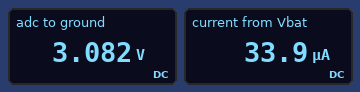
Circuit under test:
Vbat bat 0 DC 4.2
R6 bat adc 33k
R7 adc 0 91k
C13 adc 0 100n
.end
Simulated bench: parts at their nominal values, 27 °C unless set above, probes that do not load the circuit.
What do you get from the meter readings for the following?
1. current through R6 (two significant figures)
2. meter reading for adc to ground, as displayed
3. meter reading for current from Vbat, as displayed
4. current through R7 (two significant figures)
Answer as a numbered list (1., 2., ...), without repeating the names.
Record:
1. 34 µA
2. 3.082 V
3. 33.9 µA
4. 34 µA
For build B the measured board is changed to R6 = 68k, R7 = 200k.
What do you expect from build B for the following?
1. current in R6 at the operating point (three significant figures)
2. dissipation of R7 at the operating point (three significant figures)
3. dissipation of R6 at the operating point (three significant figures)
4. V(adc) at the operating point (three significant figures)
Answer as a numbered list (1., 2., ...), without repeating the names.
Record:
1. 15.7 µA
2. 49.1 µW
3. 16.7 µW
4. 3.13 V
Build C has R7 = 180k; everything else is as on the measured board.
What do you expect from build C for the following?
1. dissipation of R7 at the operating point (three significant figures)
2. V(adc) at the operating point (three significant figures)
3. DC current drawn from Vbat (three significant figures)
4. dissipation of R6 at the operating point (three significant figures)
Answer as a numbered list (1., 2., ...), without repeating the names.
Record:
1. 70.0 µW
2. 3.55 V
3. 19.7 µA
4. 12.8 µW
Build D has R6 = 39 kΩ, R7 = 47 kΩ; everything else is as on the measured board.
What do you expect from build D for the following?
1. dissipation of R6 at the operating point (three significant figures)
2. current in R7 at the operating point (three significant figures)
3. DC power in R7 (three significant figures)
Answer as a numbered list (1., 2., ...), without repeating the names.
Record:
1. 93.0 µW
2. 48.8 µA
3. 112 µW
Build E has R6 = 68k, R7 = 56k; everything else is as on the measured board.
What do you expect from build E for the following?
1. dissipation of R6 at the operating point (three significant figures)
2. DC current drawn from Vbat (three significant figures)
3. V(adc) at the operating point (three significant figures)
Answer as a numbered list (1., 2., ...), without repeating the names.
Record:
1. 78.0 µW
2. 33.9 µA
3. 1.90 V
